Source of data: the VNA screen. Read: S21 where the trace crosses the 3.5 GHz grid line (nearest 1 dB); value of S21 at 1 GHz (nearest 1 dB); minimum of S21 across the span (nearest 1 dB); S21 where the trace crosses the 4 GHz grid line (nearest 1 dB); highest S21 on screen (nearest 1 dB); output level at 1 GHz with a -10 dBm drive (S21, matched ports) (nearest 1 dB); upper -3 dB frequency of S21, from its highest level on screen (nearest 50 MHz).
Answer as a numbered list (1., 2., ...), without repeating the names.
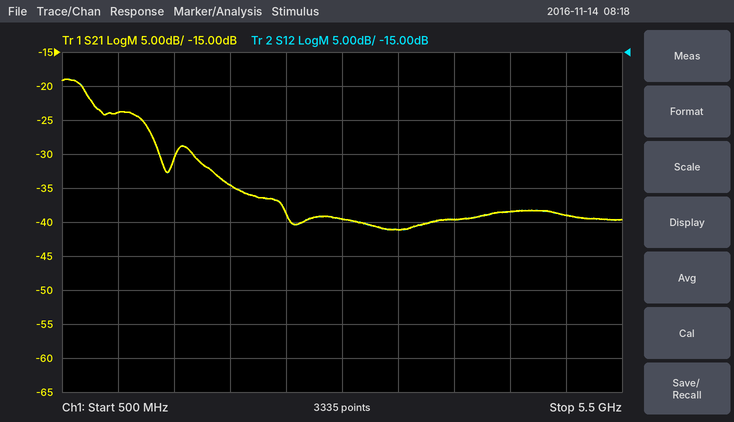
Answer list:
1. -41 dB
2. -24 dB
3. -41 dB
4. -40 dB
5. -19 dB
6. -34 dBm
7. 750 MHz
